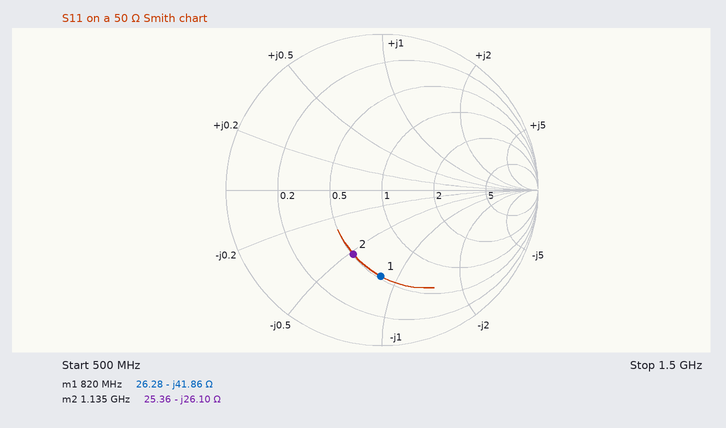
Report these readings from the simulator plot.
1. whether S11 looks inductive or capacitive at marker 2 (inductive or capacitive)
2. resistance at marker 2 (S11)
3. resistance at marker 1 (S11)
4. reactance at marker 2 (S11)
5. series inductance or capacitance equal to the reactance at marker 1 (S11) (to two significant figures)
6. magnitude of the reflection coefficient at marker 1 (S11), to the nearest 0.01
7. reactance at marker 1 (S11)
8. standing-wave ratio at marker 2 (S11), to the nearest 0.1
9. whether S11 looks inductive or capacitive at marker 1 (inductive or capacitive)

capacitive
25.36 Ω
26.28 Ω
-26.10 Ω
4.6 pF
0.55
-41.86 Ω
2.6
capacitive
